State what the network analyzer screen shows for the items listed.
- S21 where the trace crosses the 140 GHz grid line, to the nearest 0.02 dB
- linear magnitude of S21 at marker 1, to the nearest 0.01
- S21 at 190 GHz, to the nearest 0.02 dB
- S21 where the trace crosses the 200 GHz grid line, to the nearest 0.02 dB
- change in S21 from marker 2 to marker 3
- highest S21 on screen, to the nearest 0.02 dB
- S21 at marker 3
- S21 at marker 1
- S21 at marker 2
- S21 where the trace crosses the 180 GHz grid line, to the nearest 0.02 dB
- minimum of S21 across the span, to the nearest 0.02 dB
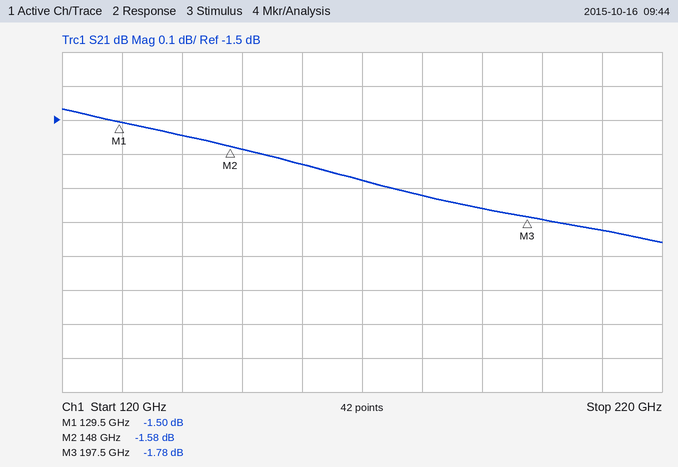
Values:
-1.54 dB
0.84
-1.76 dB
-1.80 dB
-0.20 dB
-1.46 dB
-1.78 dB
-1.50 dB
-1.58 dB
-1.72 dB
-1.86 dB
